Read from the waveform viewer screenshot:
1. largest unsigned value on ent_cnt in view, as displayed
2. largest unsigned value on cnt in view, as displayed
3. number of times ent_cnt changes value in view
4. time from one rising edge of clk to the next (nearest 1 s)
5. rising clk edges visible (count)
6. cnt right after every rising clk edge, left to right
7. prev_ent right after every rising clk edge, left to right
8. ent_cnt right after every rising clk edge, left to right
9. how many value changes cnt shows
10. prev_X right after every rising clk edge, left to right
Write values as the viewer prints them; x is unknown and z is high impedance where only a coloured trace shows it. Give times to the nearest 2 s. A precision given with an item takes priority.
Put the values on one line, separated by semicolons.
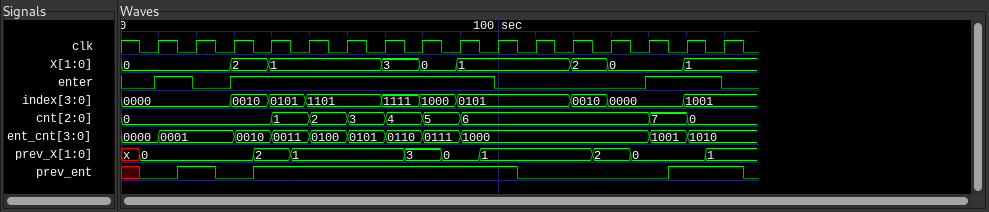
1010; 7; 10; 10 s; 16; 0, 0, 0, 1, 2, 3, 4, 5, 6, 6, 6, 6, 6, 7, 0, 0; 0 1 0 1 1 1 1 1 1 1 0 0 0 0 1 1; 0001, 0001, 0010, 0011, 0100, 0101, 0110, 0111, 1000, 1000, 1000, 1000, 1000, 1001, 1010, 1010; 8; 0, 0, 0, 2, 1, 1, 1, 3, 0, 1, 1, 1, 2, 0, 0, 1
